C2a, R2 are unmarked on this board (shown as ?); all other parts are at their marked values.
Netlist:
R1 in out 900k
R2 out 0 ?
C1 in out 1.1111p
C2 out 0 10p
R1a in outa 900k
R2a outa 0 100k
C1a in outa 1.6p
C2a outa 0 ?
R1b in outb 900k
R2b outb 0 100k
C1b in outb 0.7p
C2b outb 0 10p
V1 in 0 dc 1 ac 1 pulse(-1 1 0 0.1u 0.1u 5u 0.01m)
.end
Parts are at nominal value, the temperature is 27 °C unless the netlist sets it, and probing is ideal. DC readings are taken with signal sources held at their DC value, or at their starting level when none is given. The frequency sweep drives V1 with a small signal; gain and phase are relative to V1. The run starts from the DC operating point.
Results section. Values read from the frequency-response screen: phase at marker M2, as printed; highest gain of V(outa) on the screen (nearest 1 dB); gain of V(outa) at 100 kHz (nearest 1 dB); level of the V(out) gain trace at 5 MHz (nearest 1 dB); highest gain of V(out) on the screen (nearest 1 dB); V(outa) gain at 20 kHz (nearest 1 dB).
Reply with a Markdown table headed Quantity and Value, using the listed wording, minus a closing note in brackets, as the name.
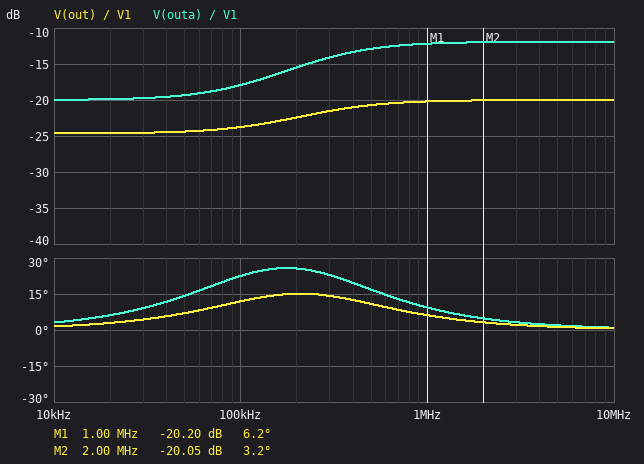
| Quantity | Value |
|---|---|
| phase at marker M2, as printed | 3.2 deg |
| highest gain of V(outa) on the screen | -12 dB |
| gain of V(outa) at 100 kHz | -18 dB |
| level of the V(out) gain trace at 5 MHz | -20 dB |
| highest gain of V(out) on the screen | -20 dB |
| V(outa) gain at 20 kHz | -20 dB |
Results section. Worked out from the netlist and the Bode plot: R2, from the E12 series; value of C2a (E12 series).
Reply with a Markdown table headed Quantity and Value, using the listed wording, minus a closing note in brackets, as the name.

| Quantity | Value |
|---|---|
| R2, from the E12 series | 56 kΩ |
| value of C2a | 4.7 pF |
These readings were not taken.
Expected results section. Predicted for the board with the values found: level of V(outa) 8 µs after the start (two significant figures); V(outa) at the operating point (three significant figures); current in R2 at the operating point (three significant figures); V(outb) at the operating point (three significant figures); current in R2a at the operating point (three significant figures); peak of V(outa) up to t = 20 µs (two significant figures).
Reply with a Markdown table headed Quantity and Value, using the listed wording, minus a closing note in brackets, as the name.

| Quantity | Value |
|---|---|
| level of V(outa) 8 µs after the start | -100 mV |
| V(outa) at the operating point | 100 mV |
| current in R2 at the operating point | 1.05 µA |
| V(outb) at the operating point | 100 mV |
| current in R2a at the operating point | 1.00 µA |
| peak of V(outa) up to t = 20 µs | 380 mV |
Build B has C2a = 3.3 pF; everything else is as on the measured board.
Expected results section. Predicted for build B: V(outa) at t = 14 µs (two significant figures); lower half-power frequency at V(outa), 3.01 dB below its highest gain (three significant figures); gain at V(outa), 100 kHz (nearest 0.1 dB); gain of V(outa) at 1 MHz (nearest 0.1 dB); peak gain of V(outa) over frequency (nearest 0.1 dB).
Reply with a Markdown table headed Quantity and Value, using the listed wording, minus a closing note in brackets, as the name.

| Quantity | Value |
|---|---|
| V(outa) at t = 14 µs | 100 mV |
| lower half-power frequency at V(outa), 3.01 dB below its highest gain | 325 kHz |
| gain at V(outa), 100 kHz | -17.7 dB |
| gain of V(outa) at 1 MHz | -10.2 dB |
| peak gain of V(outa) over frequency | -9.7 dB |
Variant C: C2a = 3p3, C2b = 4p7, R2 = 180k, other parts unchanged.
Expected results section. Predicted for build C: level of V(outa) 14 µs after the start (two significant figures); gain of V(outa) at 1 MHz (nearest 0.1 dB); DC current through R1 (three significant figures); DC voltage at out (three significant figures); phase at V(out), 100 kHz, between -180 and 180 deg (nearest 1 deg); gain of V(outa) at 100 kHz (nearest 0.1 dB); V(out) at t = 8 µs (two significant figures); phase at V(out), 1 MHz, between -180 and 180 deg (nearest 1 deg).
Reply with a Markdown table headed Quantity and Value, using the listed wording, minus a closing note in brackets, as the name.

| Quantity | Value |
|---|---|
| level of V(outa) 14 µs after the start | 100 mV |
| gain of V(outa) at 1 MHz | -10.2 dB |
| DC current through R1 | 926 nA |
| DC voltage at out | 167 mV |
| phase at V(out), 100 kHz, between -180 and 180 deg | -14 deg |
| gain of V(outa) at 100 kHz | -17.7 dB |
| V(out) at t = 8 µs | -140 mV |
| phase at V(out), 1 MHz, between -180 and 180 deg | -4 deg |
